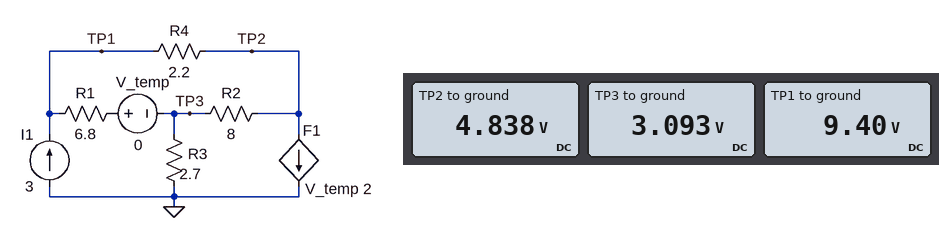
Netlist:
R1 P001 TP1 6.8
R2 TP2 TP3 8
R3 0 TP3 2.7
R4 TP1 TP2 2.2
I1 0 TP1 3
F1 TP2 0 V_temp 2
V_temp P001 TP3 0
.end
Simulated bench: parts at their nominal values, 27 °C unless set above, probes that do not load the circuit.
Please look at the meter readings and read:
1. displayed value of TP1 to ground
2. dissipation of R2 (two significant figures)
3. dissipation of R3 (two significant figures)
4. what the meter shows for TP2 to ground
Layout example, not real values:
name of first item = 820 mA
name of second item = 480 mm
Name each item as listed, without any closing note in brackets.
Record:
displayed value of TP1 to ground = 9.40 V
dissipation of R2 = 380 mW
dissipation of R3 = 3.5 W
what the meter shows for TP2 to ground = 4.838 V
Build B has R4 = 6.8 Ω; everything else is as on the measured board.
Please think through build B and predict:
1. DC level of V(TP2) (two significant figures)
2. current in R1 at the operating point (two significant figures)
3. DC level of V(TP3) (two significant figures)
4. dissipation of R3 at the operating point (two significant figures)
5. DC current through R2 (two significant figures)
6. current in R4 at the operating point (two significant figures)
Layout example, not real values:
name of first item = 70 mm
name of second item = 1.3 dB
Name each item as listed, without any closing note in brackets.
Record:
DC level of V(TP2) = -2.6 V
current in R1 at the operating point = 1.2 A
DC level of V(TP3) = 1.7 V
dissipation of R3 at the operating point = 1.1 W
DC current through R2 = 540 mA
current in R4 at the operating point = 1.8 A
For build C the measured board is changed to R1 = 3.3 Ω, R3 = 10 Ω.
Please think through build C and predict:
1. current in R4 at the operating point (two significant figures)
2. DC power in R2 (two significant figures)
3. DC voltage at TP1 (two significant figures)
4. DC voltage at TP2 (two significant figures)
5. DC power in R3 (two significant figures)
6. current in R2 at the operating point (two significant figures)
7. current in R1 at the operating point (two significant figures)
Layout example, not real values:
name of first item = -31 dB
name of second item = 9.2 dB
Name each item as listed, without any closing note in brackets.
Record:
current in R4 at the operating point = 2.0 A
DC power in R2 = 100 mW
DC voltage at TP1 = 13 V
DC voltage at TP2 = 8.4 V
DC power in R3 = 8.6 W
current in R2 at the operating point = 110 mA
current in R1 at the operating point = 1.0 A
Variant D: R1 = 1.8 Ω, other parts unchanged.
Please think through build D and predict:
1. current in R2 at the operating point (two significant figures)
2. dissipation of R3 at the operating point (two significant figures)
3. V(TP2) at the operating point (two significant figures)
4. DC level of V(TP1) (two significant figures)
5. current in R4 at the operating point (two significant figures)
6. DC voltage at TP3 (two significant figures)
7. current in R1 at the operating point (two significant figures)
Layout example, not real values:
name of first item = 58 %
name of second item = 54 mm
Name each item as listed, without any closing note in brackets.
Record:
current in R2 at the operating point = 280 mA
dissipation of R3 at the operating point = 1.8 W
V(TP2) at the operating point = -30 mV
DC level of V(TP1) = 4.2 V
current in R4 at the operating point = 1.9 A
DC voltage at TP3 = 2.2 V
current in R1 at the operating point = 1.1 A
